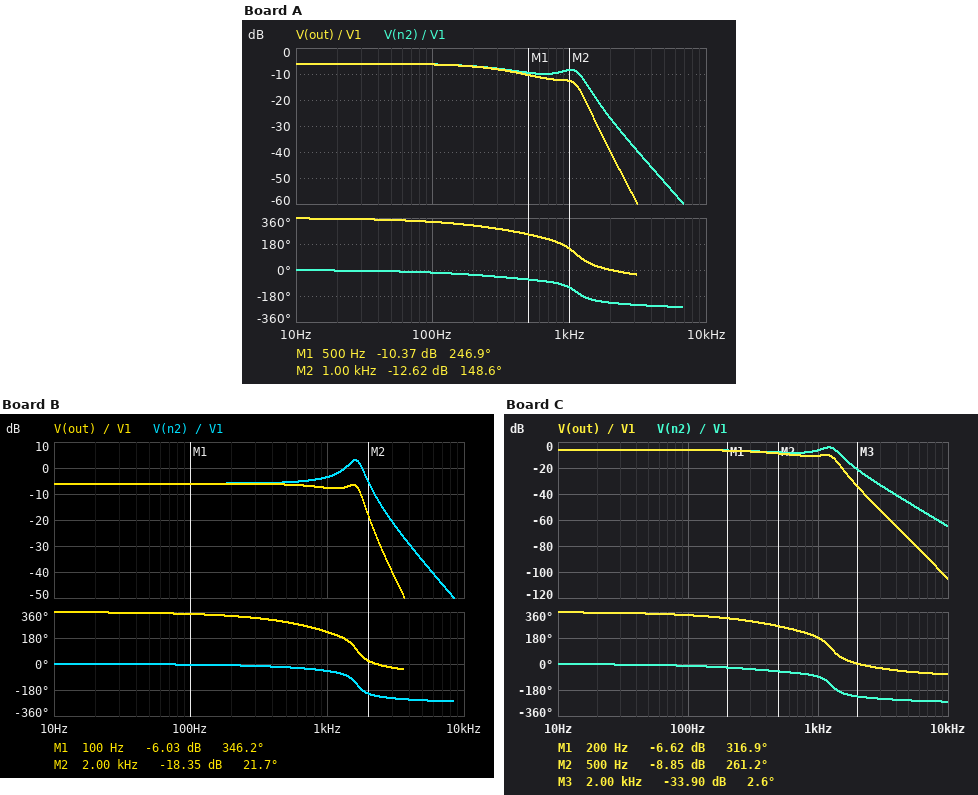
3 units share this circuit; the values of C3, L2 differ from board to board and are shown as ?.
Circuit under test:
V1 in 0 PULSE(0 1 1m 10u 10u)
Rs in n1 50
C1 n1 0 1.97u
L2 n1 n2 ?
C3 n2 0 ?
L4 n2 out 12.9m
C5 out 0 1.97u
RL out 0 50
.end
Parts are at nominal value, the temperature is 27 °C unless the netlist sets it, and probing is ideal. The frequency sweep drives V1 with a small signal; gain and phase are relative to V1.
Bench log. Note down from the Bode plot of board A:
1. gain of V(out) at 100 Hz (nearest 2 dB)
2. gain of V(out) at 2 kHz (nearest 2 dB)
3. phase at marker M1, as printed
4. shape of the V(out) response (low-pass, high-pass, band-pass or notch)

-6 dB
-40 dB
246.9 deg
low-pass
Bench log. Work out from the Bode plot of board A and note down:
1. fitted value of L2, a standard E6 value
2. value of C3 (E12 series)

47 mH
2.7 µF
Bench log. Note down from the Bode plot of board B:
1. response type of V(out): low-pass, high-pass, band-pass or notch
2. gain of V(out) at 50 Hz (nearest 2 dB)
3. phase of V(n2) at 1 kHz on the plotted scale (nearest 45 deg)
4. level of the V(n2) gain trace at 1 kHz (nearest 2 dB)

low-pass
-6 dB
-45 deg
-4 dB
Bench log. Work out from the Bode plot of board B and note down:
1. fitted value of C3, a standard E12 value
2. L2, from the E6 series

2.2 µF
10 mH
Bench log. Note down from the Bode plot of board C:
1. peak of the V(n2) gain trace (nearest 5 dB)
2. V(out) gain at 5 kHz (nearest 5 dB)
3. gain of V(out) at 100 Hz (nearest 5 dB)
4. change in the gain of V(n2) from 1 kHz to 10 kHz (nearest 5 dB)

-5 dB
-75 dB
-5 dB
-60 dB
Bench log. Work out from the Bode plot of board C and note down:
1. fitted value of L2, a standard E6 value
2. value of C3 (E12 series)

33 mH
2.2 µF
